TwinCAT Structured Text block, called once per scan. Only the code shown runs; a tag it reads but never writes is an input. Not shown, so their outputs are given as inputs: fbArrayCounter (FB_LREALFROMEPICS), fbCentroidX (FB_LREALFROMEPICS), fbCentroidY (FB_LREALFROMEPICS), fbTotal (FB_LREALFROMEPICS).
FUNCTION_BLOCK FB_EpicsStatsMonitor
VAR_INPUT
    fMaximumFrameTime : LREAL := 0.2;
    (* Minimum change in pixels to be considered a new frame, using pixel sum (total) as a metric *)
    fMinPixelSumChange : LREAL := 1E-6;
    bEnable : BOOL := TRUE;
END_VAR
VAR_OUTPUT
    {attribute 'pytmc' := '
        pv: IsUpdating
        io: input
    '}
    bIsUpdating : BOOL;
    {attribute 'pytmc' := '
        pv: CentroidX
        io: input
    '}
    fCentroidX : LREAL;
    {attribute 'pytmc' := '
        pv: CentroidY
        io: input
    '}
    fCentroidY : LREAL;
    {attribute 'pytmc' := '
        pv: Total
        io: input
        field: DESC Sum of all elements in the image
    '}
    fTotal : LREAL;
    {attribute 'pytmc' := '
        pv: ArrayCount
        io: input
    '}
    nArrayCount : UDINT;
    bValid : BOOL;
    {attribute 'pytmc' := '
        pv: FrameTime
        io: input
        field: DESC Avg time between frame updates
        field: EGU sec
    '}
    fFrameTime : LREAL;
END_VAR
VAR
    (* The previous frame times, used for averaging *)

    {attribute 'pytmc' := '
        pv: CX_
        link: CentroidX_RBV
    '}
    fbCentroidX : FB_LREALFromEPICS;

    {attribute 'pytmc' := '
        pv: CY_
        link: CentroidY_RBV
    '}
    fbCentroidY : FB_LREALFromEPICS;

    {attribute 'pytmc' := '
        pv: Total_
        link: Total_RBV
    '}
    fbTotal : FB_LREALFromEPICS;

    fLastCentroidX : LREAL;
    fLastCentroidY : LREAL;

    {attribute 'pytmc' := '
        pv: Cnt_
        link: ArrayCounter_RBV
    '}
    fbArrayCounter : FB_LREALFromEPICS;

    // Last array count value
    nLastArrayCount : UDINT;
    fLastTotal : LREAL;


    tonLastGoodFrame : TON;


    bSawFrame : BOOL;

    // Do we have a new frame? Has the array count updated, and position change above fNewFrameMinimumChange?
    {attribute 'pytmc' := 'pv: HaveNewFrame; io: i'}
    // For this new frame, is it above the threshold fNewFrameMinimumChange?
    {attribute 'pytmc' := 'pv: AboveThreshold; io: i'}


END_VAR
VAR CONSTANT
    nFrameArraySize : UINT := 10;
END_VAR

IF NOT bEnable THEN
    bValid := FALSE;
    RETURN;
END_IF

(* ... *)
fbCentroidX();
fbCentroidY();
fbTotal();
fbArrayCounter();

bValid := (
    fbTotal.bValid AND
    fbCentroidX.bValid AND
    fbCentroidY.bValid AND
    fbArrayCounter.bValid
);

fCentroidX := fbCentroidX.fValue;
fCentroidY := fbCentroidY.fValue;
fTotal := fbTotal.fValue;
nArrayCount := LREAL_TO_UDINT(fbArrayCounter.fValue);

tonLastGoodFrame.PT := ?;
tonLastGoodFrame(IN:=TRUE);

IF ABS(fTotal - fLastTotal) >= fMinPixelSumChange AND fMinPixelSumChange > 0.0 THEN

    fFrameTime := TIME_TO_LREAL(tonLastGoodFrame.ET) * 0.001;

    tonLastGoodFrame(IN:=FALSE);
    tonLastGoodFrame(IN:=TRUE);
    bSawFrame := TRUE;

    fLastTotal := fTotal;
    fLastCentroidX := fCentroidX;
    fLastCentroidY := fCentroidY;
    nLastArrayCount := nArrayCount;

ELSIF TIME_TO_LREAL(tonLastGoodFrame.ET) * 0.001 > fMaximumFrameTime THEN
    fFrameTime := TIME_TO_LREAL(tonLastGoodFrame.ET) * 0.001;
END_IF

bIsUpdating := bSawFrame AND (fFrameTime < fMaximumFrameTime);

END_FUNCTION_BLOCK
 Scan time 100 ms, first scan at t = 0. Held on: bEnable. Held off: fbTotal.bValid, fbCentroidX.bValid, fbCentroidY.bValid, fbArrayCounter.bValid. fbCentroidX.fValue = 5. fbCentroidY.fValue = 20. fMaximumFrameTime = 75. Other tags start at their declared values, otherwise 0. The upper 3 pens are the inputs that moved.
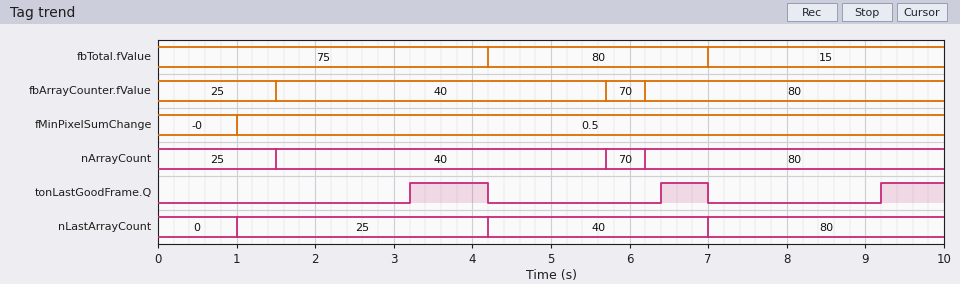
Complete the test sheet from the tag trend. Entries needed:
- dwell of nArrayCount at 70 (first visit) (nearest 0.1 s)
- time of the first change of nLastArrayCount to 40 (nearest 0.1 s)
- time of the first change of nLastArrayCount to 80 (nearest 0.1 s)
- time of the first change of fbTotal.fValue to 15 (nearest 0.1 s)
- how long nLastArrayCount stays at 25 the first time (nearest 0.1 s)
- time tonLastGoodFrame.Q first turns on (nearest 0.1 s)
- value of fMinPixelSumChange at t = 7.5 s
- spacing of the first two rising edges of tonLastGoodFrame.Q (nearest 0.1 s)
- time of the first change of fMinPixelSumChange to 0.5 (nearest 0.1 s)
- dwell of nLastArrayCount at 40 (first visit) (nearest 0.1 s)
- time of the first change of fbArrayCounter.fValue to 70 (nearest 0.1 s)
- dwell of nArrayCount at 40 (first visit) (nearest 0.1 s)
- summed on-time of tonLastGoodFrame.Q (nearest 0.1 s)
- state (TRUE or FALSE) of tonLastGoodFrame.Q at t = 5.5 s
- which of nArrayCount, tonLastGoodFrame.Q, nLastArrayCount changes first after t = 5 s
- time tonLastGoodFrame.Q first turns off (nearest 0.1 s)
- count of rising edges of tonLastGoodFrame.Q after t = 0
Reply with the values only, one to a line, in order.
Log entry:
0.5 s
4.2 s
7.0 s
7.0 s
3.2 s
3.2 s
0.5
3.2 s
1.0 s
2.8 s
5.7 s
4.2 s
2.4 s
FALSE
nArrayCount
4.2 s
3
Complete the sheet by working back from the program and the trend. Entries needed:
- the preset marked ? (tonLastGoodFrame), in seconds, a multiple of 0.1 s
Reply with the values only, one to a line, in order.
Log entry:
2.2 s
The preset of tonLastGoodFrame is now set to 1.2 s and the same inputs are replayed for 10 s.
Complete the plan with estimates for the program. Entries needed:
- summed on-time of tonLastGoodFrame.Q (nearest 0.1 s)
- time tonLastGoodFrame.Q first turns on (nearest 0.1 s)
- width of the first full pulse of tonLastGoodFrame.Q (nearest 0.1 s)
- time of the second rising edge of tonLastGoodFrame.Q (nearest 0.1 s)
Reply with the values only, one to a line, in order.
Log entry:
5.4 s
2.2 s
2.0 s
5.4 s
